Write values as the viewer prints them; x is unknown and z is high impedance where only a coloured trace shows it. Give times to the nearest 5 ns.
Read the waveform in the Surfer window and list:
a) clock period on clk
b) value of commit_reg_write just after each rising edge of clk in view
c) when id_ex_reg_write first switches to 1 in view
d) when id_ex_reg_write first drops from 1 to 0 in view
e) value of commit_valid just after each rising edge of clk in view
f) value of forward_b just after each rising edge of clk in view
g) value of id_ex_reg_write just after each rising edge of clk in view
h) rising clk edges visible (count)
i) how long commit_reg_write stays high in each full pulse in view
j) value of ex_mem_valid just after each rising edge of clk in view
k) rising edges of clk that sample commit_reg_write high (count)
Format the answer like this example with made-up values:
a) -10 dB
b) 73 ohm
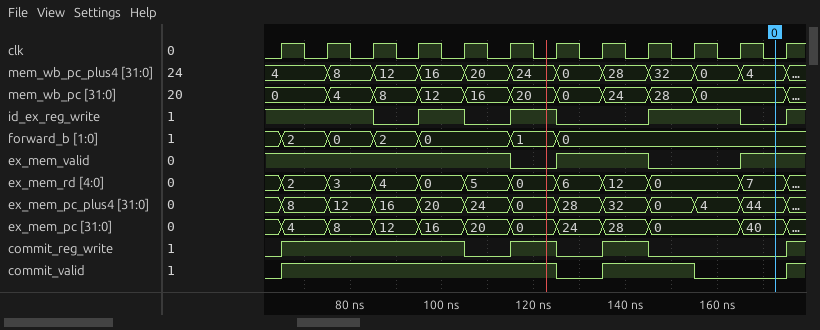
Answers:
a) 10 ns
b) 1 1 1 1 0 1 0 1 0 0 0 1
c) 95 ns
d) 85 ns
e) 1 1 1 1 1 1 0 1 1 0 0 1
f) 2, 0, 2, 0, 0, 1, 0, 0, 0, 0, 0, 0
g) 1 1 0 1 0 1 0 0 1 1 0 1
h) 12
i) 40 ns, 10 ns, 10 ns
j) 1 1 1 1 1 0 1 1 0 0 1 1
k) 6
